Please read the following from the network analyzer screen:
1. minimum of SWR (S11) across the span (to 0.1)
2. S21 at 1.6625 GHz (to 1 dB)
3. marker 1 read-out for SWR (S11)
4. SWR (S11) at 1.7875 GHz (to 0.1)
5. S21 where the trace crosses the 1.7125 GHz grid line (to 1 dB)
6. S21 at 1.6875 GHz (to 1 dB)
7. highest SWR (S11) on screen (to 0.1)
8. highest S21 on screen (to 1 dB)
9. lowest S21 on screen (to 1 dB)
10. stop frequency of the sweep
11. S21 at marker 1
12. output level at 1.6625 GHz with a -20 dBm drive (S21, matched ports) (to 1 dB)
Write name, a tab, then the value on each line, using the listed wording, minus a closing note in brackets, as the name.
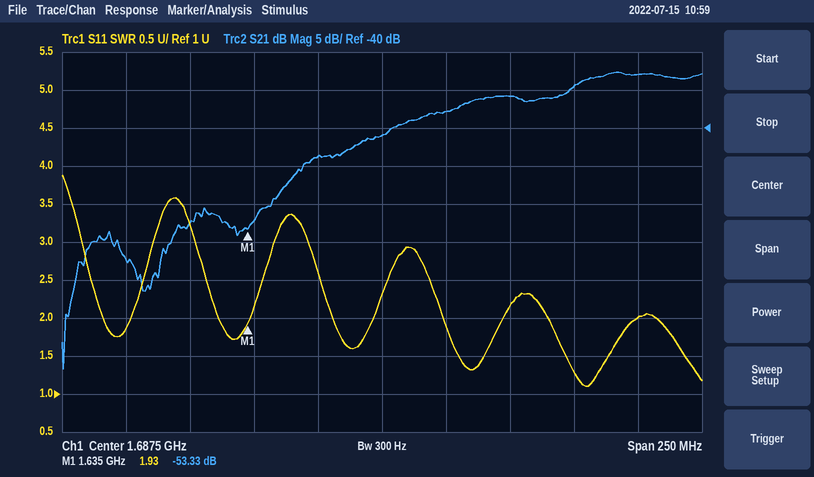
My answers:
minimum of SWR (S11) across the span	1.1
S21 at 1.6625 GHz	-44 dB
marker 1 read-out for SWR	1.93
SWR (S11) at 1.7875 GHz	2.0
S21 where the trace crosses the 1.7125 GHz grid line	-38 dB
S21 at 1.6875 GHz	-41 dB
highest SWR (S11) on screen	3.9
highest S21 on screen	-33 dB
lowest S21 on screen	-72 dB
stop frequency of the sweep	1.8125 GHz
S21 at marker 1	-53.33 dB
output level at 1.6625 GHz with a -20 dBm drive (S21, matched ports)	-64 dBm
